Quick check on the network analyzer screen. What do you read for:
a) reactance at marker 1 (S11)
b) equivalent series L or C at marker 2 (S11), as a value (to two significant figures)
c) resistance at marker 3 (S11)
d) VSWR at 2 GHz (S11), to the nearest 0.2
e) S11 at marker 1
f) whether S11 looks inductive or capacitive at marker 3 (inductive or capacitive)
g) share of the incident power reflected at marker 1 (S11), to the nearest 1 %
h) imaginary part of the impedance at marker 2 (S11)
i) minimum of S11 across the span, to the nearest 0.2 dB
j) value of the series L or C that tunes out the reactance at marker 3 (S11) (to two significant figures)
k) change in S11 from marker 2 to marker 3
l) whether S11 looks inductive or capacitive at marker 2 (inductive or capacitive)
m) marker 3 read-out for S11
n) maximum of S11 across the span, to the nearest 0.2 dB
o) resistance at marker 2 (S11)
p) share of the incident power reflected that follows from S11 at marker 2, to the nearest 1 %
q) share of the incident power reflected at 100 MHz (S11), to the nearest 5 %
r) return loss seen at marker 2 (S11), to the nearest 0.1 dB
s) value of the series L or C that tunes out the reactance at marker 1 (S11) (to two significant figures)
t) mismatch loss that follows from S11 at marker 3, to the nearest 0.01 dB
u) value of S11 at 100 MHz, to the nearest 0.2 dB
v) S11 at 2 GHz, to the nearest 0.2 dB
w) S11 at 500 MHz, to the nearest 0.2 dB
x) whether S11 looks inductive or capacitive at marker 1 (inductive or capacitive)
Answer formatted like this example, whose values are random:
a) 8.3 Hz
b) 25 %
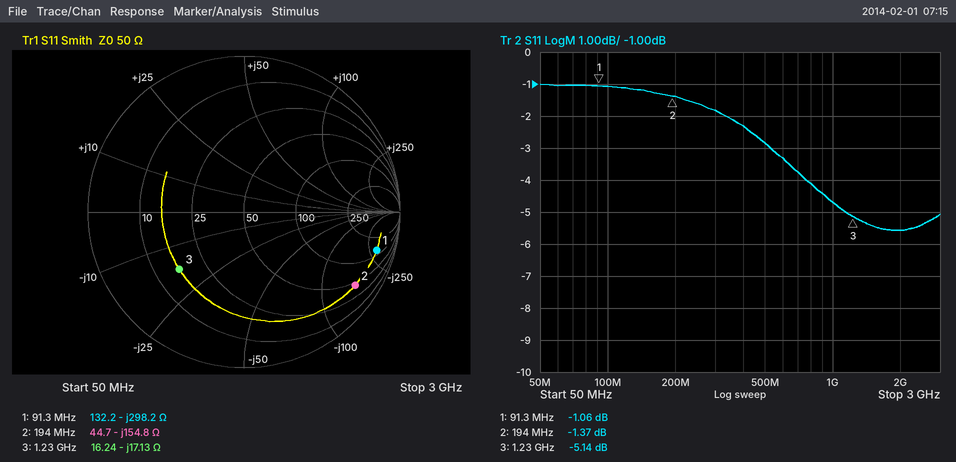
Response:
a) -298.2 Ω
b) 5.3 pF
c) 16.24 Ω
d) 3.2
e) -1.06 dB
f) capacitive
g) 78 %
h) -154.8 Ω
i) -5.6 dB
j) 2.2 nH
k) -3.77 dB
l) capacitive
m) -5.14 dB
n) -1.0 dB
o) 44.7 Ω
p) 73 %
q) 80 %
r) 1.4 dB
s) 520 nH
t) 1.59 dB
u) -1.0 dB
v) -5.6 dB
w) -2.8 dB
x) capacitive
